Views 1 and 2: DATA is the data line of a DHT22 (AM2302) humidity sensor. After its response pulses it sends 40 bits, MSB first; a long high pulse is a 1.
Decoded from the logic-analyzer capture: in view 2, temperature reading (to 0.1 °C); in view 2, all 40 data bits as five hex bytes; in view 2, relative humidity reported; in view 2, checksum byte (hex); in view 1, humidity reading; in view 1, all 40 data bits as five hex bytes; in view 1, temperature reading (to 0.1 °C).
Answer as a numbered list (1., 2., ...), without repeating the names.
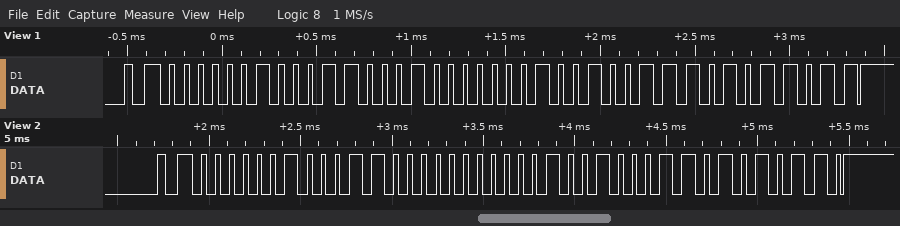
1. 29.1 °C
2. 02 30 01 23 56
3. 56.0 %
4. 0x56
5. 56.1 %
6. 02 31 01 27 5B
7. 29.5 °C
